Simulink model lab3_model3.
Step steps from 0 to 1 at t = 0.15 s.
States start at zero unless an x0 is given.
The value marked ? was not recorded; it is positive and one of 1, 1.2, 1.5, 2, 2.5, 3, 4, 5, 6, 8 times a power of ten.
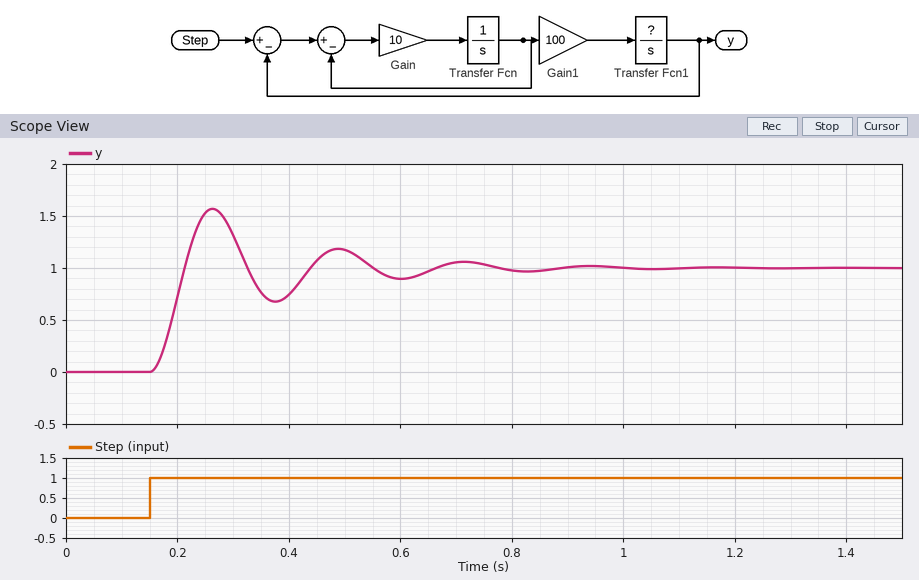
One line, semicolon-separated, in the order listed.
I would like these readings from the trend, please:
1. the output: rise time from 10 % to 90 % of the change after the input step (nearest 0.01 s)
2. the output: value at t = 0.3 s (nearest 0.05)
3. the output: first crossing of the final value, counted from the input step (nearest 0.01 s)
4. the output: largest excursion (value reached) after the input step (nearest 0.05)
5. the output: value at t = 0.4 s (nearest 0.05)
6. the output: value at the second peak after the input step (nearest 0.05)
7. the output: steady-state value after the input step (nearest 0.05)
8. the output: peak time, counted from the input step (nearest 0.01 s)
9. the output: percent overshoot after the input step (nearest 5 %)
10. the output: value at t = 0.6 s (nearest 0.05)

0.04 s; 1.30; 0.06 s; 1.55; 0.75; 1.20; 1.00; 0.11 s; 55 %; 0.90
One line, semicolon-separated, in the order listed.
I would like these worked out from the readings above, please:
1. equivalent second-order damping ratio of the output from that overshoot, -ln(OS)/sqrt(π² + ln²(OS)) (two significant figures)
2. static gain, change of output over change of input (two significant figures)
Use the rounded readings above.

0.19; 1.0
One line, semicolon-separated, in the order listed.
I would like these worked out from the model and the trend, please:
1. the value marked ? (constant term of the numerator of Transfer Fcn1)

0.8
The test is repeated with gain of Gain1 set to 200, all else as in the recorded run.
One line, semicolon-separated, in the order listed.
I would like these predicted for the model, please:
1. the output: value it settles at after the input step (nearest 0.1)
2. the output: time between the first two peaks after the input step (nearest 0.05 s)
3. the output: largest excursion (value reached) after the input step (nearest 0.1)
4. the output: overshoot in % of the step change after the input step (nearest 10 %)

1.0; 0.15 s; 1.7; 70 %
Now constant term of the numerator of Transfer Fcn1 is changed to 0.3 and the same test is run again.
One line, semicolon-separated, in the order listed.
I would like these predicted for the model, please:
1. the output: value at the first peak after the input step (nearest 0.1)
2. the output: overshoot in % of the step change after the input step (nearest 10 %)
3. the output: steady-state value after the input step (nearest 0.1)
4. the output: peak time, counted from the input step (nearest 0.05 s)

1.4; 40 %; 1.0; 0.20 s
